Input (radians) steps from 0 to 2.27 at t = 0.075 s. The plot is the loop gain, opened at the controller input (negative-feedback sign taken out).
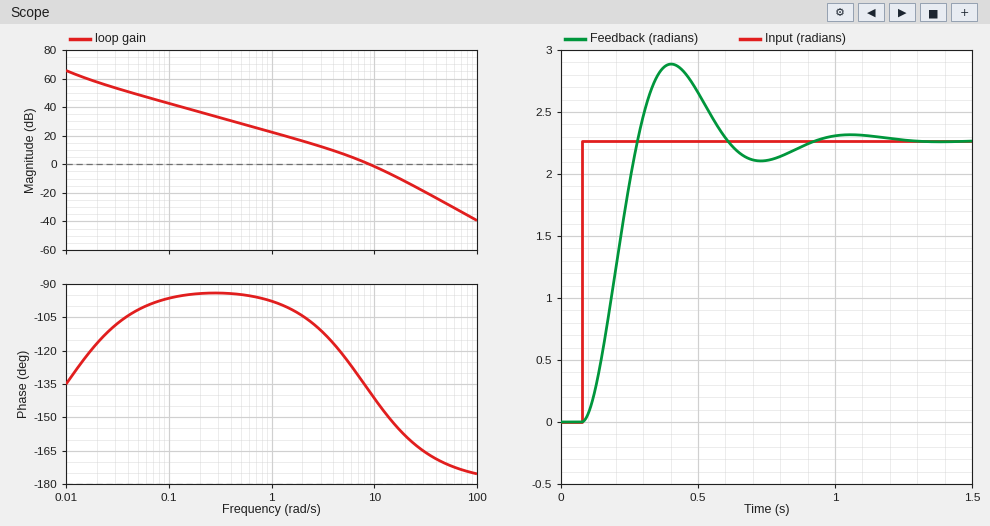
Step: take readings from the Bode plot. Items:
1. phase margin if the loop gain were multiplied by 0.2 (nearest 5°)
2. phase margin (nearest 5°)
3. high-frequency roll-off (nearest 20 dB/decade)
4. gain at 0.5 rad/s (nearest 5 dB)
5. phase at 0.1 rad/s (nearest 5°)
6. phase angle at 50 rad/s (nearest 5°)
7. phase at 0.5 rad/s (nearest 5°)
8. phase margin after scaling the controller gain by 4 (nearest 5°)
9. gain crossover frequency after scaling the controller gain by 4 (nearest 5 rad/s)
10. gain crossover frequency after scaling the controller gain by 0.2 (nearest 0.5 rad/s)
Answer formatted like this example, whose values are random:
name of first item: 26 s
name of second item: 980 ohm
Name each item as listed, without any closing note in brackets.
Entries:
phase margin if the loop gain were multiplied by 0.2: 70°
phase margin: 40°
high-frequency roll-off: -40 dB/decade
gain at 0.5 rad/s: 30 dB
phase at 0.1 rad/s: -95°
phase angle at 50 rad/s: -170°
phase at 0.5 rad/s: -95°
phase margin after scaling the controller gain by 4: 20°
gain crossover frequency after scaling the controller gain by 4: 20 rad/s
gain crossover frequency after scaling the controller gain by 0.2: 2.5 rad/s
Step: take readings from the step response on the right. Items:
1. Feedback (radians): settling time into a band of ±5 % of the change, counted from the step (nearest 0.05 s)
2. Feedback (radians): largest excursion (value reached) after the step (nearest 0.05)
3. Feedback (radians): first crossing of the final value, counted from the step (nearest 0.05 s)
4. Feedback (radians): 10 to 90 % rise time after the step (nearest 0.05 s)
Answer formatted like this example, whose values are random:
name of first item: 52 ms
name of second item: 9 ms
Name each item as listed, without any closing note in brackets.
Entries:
Feedback (radians): settling time into a band of ±5 % of the change, counted from the step: 0.75 s
Feedback (radians): largest excursion (value reached) after the step: 2.90
Feedback (radians): first crossing of the final value, counted from the step: 0.20 s
Feedback (radians): 10 to 90 % rise time after the step: 0.15 s
